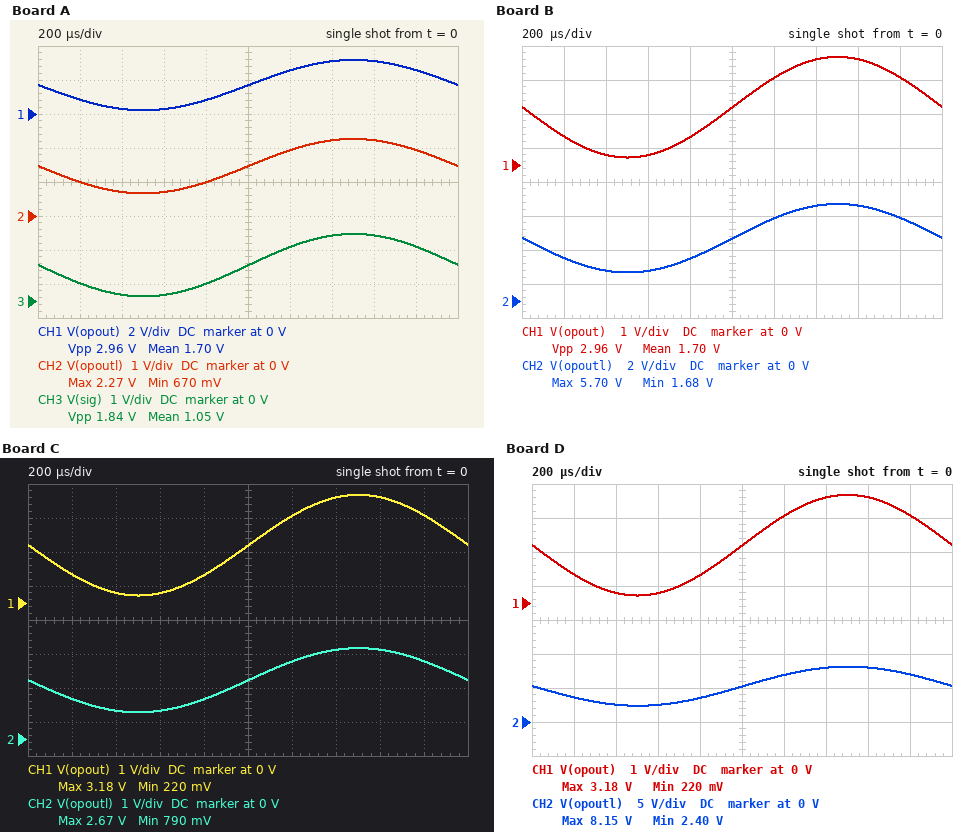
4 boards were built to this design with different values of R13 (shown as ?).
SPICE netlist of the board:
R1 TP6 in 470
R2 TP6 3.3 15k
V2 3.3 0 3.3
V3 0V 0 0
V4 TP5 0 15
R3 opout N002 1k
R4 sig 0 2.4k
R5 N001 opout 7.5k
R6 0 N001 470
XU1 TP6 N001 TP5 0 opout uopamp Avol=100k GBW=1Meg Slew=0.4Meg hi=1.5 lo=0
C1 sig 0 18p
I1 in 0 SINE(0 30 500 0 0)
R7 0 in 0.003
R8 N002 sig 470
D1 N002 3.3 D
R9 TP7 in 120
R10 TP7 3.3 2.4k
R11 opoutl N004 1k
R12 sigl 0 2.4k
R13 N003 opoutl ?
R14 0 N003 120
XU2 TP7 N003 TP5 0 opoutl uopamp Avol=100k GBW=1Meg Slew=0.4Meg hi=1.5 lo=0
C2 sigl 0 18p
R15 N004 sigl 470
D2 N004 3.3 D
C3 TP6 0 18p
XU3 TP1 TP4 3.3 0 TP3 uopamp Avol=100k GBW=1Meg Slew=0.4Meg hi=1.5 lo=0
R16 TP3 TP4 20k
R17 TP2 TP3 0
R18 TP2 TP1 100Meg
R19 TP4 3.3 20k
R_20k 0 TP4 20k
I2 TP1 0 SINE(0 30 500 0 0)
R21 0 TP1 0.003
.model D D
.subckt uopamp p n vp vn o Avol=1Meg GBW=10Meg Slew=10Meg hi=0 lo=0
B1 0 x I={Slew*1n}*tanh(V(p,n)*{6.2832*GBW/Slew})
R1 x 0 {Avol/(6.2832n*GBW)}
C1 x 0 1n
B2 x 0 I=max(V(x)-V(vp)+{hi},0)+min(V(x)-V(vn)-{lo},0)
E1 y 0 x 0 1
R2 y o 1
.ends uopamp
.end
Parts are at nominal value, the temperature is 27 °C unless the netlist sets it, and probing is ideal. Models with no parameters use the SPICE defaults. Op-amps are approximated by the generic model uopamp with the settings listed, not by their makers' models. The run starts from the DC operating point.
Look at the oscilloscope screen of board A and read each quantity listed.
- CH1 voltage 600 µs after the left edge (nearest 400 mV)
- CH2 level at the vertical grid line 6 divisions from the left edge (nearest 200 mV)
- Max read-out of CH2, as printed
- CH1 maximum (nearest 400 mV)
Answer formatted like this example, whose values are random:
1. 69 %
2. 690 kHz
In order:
1. 400 mV
2. 2.0 V
3. 2.27 V
4. 3.2 V
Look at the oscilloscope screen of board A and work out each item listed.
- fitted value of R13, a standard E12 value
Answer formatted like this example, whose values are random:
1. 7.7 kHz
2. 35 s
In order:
1. 1 kΩ
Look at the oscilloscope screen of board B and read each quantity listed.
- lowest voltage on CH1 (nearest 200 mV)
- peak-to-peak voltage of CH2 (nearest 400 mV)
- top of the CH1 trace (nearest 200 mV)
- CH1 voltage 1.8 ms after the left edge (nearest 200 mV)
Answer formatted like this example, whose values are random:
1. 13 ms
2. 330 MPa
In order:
1. 200 mV
2. 4.0 V
3. 3.2 V
4. 2.6 V
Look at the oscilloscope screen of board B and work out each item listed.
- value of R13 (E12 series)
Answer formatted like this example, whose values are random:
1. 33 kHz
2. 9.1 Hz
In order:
1. 2.7 kΩ
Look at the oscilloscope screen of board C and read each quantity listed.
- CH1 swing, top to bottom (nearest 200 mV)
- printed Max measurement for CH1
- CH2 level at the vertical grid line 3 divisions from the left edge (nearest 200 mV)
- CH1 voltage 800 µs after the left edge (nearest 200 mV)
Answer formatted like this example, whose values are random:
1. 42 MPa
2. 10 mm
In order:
1. 3.0 V
2. 3.18 V
3. 800 mV
4. 800 mV
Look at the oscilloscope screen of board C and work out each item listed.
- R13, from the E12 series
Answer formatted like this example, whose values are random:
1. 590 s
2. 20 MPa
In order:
1. 1.2 kΩ
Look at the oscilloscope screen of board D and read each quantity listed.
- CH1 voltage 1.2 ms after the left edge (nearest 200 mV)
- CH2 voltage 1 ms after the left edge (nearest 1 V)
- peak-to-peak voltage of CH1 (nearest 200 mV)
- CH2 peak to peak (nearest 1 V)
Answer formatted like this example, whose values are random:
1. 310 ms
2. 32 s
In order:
1. 2.6 V
2. 5 V
3. 3.0 V
4. 6 V
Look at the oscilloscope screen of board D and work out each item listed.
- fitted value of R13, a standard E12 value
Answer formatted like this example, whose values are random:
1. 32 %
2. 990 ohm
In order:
1. 3.9 kΩ
